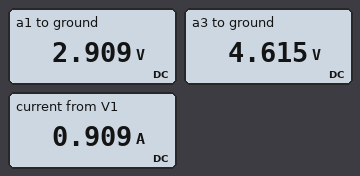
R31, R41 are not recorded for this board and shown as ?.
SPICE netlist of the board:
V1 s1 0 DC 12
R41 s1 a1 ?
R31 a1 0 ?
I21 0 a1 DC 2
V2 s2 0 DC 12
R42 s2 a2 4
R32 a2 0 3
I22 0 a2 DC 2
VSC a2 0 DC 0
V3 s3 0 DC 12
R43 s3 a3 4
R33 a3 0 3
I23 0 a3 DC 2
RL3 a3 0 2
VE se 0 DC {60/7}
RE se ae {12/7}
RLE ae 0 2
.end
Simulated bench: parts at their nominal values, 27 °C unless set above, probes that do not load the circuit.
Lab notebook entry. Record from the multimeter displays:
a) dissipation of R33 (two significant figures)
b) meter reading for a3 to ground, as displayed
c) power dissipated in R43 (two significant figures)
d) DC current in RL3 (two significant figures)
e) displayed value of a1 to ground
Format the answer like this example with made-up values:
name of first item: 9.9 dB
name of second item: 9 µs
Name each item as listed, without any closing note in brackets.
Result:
dissipation of R33: 7.1 W
meter reading for a3 to ground, as displayed: 4.615 V
power dissipated in R43: 14 W
DC current in RL3: 2.3 A
displayed value of a1 to ground: 2.909 V
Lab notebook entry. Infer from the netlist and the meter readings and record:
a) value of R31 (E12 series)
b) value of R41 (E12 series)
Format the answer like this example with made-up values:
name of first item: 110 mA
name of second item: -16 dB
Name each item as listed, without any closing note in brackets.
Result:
value of R31: 1 Ω
value of R41: 10 Ω
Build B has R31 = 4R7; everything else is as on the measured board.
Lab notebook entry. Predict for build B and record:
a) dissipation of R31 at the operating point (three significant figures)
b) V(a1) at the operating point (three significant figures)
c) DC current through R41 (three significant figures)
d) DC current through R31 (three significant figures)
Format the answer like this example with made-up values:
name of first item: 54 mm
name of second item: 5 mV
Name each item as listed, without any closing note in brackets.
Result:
dissipation of R31 at the operating point: 22.3 W
V(a1) at the operating point: 10.2 V
DC current through R41: 177 mA
DC current through R31: 2.18 A
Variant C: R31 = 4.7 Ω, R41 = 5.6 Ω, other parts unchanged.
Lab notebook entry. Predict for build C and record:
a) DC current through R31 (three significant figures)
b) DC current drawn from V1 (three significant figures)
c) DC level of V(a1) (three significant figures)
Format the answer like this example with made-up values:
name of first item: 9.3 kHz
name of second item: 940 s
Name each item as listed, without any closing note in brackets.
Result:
DC current through R31: 2.25 A
DC current drawn from V1: 252 mA
DC level of V(a1): 10.6 V
